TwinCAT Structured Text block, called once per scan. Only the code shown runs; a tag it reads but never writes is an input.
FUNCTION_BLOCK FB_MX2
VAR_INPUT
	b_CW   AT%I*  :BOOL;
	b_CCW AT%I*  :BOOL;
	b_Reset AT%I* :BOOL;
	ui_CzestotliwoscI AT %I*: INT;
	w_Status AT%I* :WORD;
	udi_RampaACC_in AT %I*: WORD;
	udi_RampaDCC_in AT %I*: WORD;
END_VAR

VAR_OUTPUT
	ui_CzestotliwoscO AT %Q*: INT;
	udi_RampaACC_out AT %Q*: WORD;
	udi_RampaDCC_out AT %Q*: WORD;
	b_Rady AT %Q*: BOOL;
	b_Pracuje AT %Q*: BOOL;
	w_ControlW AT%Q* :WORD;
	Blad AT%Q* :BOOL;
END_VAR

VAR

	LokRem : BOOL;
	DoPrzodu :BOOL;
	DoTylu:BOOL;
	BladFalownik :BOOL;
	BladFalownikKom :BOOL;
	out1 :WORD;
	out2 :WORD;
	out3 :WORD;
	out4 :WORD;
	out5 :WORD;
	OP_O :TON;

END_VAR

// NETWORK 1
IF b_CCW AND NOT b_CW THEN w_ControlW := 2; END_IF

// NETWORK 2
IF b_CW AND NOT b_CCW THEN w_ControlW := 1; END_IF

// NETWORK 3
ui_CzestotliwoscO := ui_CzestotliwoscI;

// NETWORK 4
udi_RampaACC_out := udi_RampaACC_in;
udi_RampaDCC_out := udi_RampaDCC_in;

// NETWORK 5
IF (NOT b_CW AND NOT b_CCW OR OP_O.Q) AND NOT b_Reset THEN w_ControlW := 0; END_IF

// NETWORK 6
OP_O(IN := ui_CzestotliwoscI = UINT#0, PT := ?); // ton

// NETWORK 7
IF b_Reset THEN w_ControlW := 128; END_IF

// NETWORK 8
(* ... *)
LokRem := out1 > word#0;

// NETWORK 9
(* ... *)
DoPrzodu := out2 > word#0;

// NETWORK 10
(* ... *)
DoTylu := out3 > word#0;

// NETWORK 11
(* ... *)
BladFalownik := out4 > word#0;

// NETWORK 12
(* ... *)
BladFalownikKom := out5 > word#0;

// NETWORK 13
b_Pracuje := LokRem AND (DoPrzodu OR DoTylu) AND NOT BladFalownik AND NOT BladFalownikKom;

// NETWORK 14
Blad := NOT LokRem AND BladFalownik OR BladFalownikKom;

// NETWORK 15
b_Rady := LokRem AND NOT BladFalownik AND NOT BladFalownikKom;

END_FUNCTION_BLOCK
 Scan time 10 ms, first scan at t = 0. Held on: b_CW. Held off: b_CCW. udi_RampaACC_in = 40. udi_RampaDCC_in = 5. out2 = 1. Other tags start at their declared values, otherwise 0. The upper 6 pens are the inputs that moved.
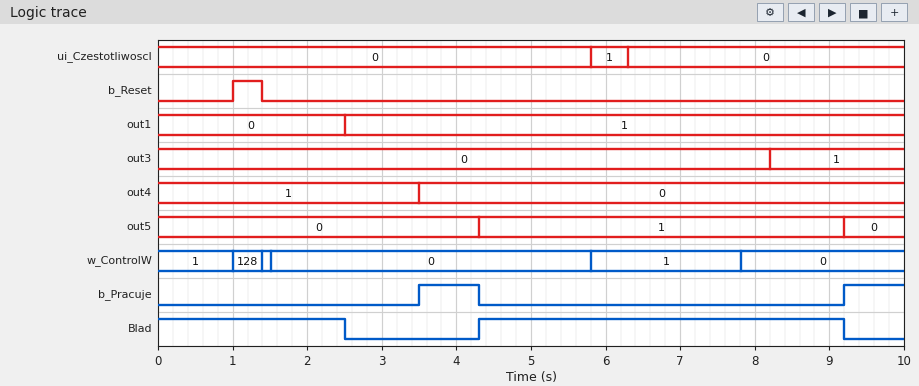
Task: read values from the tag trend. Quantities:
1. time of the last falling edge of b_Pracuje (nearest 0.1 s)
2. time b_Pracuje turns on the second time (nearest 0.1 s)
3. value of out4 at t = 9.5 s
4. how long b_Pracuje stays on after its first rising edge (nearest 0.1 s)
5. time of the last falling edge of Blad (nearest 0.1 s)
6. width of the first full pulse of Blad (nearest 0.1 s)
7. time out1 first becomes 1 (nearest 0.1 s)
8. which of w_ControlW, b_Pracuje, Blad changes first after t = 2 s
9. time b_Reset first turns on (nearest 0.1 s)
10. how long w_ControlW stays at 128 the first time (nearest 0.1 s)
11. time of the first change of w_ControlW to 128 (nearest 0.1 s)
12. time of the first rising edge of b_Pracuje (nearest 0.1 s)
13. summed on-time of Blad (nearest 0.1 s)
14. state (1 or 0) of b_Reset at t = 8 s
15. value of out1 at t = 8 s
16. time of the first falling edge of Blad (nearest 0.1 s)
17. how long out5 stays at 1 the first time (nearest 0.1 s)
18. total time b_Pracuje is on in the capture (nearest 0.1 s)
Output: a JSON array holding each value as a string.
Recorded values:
["4.3 s", "9.2 s", "0", "0.8 s", "9.2 s", "4.9 s", "2.5 s", "Blad", "1.0 s", "0.4 s", "1.0 s", "3.5 s", "7.4 s", "0", "1", "2.5 s", "4.9 s", "1.6 s"]
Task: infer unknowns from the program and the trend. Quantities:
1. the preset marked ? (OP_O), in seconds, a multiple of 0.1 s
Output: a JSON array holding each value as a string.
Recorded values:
["1.5 s"]
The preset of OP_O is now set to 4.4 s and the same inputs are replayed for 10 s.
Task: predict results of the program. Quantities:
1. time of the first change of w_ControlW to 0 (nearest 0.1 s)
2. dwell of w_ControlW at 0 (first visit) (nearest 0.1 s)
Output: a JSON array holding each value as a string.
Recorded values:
["4.4 s", "1.4 s"]
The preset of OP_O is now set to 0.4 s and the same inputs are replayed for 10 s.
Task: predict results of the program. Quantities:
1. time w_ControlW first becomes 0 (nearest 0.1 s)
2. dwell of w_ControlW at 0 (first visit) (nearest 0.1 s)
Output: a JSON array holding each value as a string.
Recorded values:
["0.4 s", "0.6 s"]
